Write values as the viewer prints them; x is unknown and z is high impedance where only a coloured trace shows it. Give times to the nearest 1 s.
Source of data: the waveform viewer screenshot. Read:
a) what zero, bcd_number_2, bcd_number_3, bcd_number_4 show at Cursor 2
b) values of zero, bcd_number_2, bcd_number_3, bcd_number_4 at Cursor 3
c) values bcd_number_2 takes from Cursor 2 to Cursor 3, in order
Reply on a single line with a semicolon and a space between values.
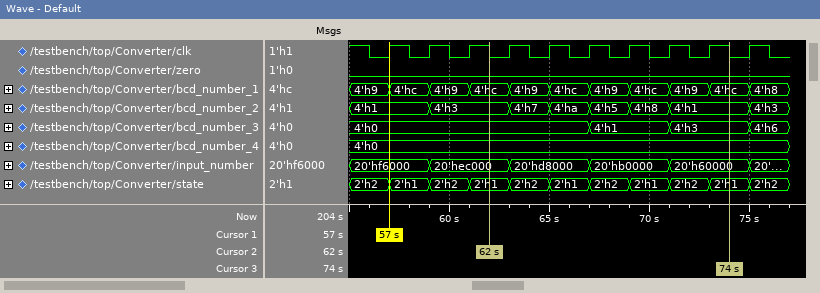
zero=0, bcd_number_2=4'h3, bcd_number_3=4'h0, bcd_number_4=4'h0; zero=0, bcd_number_2=4'h1, bcd_number_3=4'h3, bcd_number_4=4'h0; 4'h3, 4'h7, 4'ha, 4'h5, 4'h8, 4'h1
